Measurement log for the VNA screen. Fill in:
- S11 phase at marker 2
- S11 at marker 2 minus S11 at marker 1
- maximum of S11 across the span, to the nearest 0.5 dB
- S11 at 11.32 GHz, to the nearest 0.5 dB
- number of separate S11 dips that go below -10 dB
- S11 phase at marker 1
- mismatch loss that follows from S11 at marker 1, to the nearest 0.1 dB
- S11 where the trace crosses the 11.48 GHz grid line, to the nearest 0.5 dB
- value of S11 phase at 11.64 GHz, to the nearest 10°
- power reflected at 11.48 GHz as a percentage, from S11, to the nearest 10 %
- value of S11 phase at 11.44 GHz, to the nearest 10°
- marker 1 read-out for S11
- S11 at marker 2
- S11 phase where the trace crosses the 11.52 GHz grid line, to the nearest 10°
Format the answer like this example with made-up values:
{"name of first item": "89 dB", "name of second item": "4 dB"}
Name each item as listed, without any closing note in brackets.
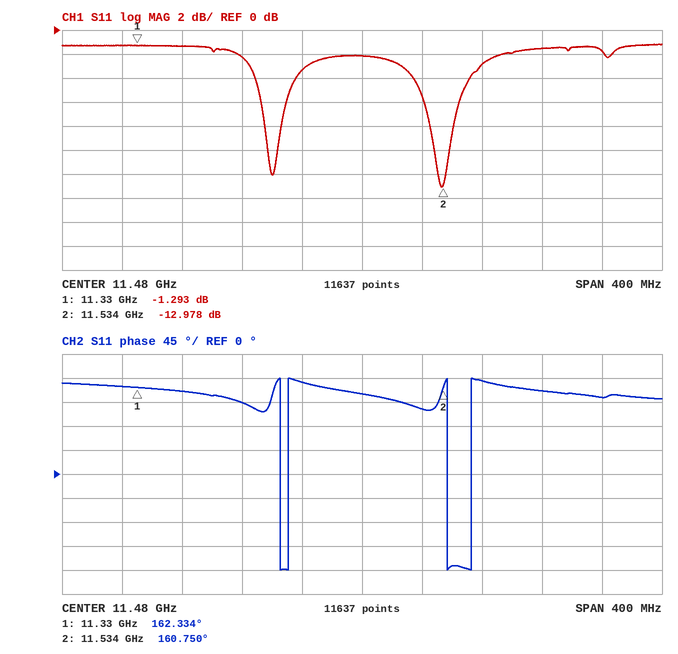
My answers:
{"S11 phase at marker 2": "160.750°", "S11 at marker 2 minus S11 at marker 1": "-11.685 dB", "maximum of S11 across the span, to the nearest 0.5 dB": "-1.0 dB", "S11 at 11.32 GHz, to the nearest 0.5 dB": "-1.5 dB", "number of separate S11 dips that go below -10 dB": "2", "S11 phase at marker 1": "162.334°", "mismatch loss that follows from S11 at marker 1, to the nearest 0.1 dB": "5.9 dB", "S11 where the trace crosses the 11.48 GHz grid line, to the nearest 0.5 dB": "-2.0 dB", "value of S11 phase at 11.64 GHz, to the nearest 10°": "140°", "power reflected at 11.48 GHz as a percentage, from S11, to the nearest 10 %": "60 %", "value of S11 phase at 11.44 GHz, to the nearest 10°": "170°", "marker 1 read-out for S11": "-1.293 dB", "S11 at marker 2": "-12.978 dB", "S11 phase where the trace crosses the 11.52 GHz grid line, to the nearest 10°": "120°"}
